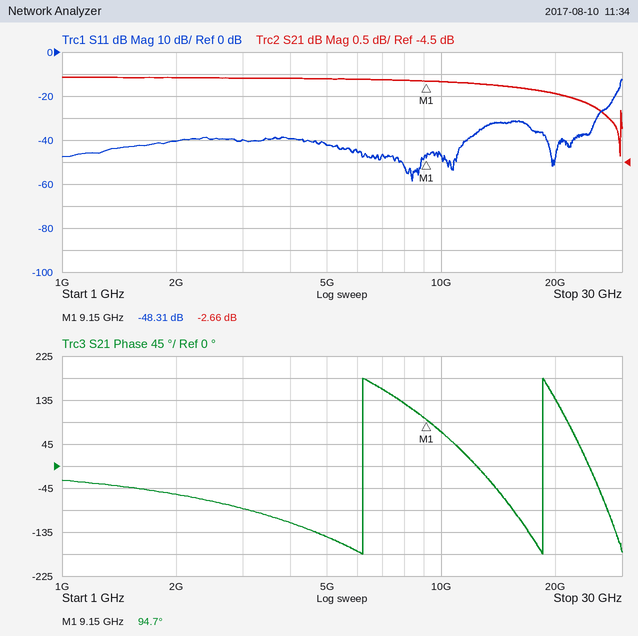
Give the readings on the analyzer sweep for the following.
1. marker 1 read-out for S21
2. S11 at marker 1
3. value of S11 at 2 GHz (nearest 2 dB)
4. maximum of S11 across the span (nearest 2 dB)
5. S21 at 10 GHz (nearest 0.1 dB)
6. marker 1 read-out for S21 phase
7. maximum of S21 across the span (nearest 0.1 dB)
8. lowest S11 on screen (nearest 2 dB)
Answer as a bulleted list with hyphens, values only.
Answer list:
- -2.66 dB
- -48.31 dB
- -40 dB
- -12 dB
- -2.7 dB
- 94.7°
- -2.6 dB
- -58 dB
